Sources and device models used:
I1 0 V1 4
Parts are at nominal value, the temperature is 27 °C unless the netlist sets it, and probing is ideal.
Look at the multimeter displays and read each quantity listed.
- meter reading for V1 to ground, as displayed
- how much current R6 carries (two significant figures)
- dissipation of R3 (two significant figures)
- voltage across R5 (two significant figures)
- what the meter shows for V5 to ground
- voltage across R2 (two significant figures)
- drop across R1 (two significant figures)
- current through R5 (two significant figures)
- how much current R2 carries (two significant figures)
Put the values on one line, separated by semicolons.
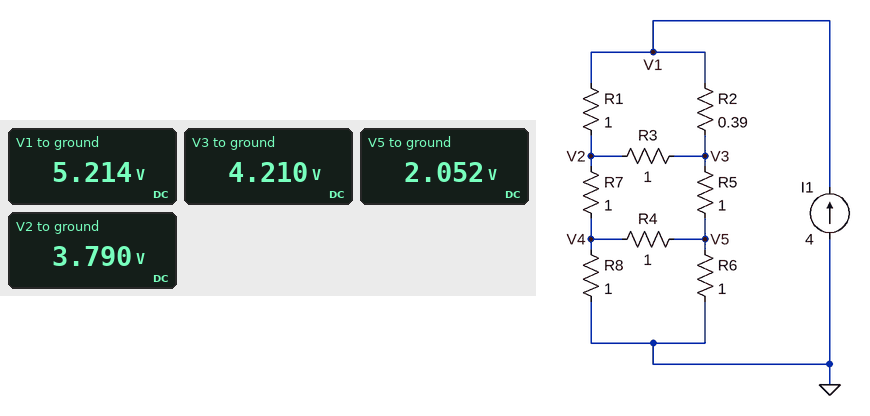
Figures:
5.214 V; 2.1 A; 180 mW; 2.2 V; 2.052 V; 1.0 V; 1.4 V; 2.2 A; 2.6 A
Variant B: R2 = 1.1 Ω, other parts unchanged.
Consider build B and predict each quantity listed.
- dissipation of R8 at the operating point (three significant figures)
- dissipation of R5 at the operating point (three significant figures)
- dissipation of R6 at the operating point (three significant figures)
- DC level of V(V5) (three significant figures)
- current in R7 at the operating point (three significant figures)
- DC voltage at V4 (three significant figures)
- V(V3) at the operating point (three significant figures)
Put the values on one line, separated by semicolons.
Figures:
4.03 W; 3.92 W; 3.97 W; 1.99 V; 2.02 A; 2.01 V; 3.97 V
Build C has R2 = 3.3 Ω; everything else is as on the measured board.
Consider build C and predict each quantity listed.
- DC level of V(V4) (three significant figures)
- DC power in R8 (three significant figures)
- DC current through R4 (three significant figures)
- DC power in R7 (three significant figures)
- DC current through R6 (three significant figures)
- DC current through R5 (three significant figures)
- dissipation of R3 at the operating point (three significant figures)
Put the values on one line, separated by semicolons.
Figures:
2.08 V; 4.34 W; 166 mA; 5.06 W; 1.92 A; 1.75 A; 443 mW
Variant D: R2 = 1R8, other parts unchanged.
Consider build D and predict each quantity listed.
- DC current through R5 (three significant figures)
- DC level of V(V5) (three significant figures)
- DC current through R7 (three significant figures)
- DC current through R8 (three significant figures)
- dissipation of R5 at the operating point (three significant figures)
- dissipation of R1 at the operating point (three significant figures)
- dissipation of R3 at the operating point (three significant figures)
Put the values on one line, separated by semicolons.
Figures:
1.88 A; 1.96 V; 2.12 A; 2.04 A; 3.52 W; 6.02 W; 109 mW
